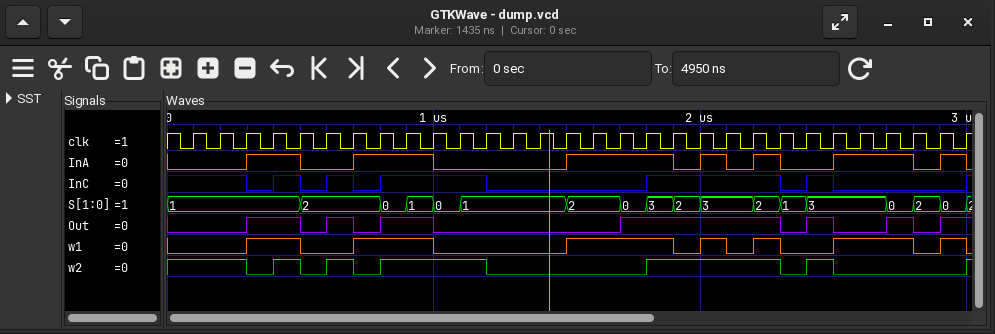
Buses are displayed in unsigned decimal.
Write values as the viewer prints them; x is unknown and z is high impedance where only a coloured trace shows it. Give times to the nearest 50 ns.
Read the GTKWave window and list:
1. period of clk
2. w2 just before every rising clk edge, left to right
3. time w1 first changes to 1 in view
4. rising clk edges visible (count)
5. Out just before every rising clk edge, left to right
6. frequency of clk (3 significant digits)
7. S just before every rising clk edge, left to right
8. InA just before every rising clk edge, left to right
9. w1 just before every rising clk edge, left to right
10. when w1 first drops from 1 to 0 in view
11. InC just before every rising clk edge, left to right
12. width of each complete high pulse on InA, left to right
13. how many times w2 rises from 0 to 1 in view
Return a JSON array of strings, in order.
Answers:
["100 ns", "1 1 1 0 1 0 1 0 1 1 1 1 0 0 0 0 0 0 1 1 1 1 1 0 1 0 0 0 0 0", "300 ns", "30", "0 0 0 1 1 0 1 0 1 1 0 0 0 0 0 0 0 1 1 1 1 1 1 0 1 0 0 1 0 1", "10.0 MHz", "1, 1, 1, 1, 1, 2, 2, 2, 0, 1, 0, 1, 1, 1, 1, 2, 2, 0, 3, 2, 3, 3, 2, 1, 3, 3, 3, 0, 2, 0", "0 0 0 1 1 0 0 1 1 1 0 0 0 0 0 1 1 1 1 0 1 0 1 0 0 1 1 1 0 1", "0 0 0 1 1 0 0 1 1 1 0 0 0 0 0 1 1 1 1 0 1 0 1 0 0 1 1 1 0 1", "500 ns", "1 1 1 0 1 0 1 0 1 1 1 1 0 0 0 0 0 0 1 1 1 1 1 0 1 0 0 0 0 0", "200 ns, 300 ns, 400 ns, 100 ns, 100 ns, 300 ns, 100 ns", "6"]
